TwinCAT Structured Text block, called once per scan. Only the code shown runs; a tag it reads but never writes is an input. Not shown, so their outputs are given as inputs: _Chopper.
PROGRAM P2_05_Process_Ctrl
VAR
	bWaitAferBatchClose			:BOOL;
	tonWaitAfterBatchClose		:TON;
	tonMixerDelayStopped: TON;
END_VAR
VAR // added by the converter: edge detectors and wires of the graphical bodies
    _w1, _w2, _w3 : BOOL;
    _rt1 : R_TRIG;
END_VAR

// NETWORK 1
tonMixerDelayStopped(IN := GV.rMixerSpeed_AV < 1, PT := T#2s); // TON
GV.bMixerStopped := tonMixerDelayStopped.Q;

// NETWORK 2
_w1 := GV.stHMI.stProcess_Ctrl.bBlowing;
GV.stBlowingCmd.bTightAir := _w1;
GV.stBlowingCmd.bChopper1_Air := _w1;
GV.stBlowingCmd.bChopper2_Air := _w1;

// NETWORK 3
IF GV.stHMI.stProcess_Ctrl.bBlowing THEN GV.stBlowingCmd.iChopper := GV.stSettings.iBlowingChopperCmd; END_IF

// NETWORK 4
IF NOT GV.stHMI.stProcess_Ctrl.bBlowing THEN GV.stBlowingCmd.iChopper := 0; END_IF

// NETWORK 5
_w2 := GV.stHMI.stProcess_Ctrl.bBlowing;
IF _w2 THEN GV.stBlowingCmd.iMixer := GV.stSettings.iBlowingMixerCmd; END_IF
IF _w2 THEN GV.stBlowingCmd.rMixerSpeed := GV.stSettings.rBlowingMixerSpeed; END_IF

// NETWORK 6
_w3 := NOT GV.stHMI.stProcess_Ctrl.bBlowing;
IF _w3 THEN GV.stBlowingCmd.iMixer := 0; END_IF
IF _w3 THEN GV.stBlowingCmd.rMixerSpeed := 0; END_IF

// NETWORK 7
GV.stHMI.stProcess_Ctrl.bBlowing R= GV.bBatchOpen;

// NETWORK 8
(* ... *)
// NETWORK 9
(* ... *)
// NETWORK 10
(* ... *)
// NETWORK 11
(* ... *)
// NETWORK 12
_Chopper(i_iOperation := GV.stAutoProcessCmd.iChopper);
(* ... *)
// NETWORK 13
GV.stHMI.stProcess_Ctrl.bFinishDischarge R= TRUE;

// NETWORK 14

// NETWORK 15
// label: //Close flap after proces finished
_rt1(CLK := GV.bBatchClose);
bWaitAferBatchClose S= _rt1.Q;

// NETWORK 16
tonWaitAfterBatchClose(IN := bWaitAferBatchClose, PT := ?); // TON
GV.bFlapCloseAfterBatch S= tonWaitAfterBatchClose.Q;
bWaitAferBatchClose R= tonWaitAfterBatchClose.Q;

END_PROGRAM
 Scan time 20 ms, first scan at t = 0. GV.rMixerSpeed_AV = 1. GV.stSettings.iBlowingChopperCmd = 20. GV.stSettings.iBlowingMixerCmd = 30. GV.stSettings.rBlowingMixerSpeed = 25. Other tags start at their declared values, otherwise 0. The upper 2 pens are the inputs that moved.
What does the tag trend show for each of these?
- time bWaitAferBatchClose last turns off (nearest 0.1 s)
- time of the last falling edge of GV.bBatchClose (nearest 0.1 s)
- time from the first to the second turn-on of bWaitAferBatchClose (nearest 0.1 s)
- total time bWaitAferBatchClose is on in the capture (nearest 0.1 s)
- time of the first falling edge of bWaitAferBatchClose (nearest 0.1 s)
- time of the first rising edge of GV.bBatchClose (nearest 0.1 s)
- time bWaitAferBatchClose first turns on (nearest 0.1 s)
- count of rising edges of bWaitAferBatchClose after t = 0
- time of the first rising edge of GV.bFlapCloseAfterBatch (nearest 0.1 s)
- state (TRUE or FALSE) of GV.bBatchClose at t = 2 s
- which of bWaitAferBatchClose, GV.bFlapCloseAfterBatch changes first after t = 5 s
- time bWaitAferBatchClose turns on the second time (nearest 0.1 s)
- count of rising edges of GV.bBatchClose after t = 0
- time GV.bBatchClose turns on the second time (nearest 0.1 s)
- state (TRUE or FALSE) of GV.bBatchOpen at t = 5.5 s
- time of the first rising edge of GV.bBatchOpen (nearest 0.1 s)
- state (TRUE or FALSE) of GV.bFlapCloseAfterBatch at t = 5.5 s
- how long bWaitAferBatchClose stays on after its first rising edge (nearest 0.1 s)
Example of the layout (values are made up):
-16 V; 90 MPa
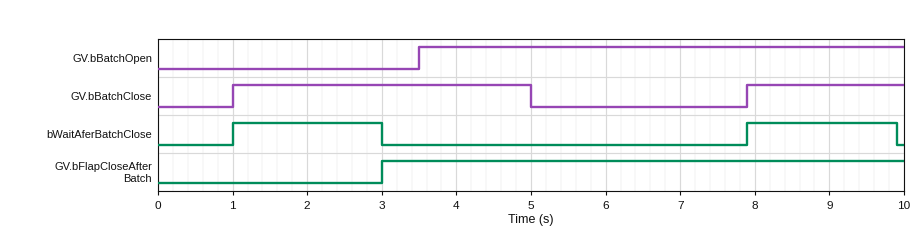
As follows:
9.9 s; 5.0 s; 6.9 s; 4.0 s; 3.0 s; 1.0 s; 1.0 s; 2; 3.0 s; TRUE; bWaitAferBatchClose; 7.9 s; 2; 7.9 s; TRUE; 3.5 s; TRUE; 2.0 s
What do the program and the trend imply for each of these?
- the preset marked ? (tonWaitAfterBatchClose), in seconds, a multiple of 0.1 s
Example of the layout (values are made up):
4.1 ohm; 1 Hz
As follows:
2.0 s
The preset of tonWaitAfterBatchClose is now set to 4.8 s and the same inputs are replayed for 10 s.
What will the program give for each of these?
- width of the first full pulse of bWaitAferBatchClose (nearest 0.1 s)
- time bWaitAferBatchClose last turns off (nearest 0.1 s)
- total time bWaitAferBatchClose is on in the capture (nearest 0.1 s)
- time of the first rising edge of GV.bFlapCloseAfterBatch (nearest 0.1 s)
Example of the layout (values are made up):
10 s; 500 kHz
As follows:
4.8 s; 5.8 s; 6.9 s; 5.8 s
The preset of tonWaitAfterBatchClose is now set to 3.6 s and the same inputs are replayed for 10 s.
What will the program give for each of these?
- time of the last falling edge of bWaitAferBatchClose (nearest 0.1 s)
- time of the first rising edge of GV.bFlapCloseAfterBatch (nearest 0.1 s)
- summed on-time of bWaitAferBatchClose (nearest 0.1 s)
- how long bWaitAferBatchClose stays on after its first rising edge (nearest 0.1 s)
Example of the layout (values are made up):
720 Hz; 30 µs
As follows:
4.6 s; 4.6 s; 5.7 s; 3.6 s
